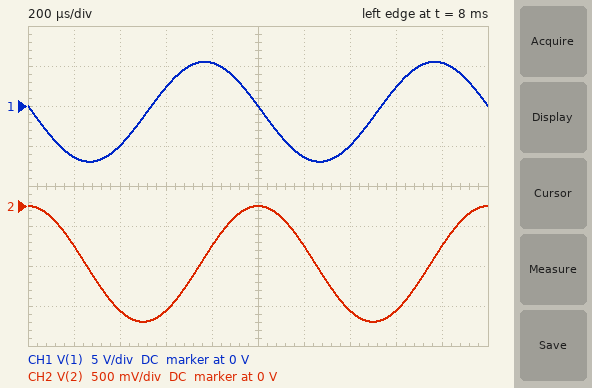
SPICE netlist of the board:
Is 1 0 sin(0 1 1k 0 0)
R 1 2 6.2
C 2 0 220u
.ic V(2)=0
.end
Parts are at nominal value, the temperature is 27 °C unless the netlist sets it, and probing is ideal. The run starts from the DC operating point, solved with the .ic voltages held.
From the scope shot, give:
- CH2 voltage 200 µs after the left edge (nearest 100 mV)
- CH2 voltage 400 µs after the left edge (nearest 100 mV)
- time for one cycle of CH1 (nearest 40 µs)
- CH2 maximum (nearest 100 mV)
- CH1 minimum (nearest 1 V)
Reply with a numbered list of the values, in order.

1. -500 mV
2. -1.3 V
3. 1.00 ms
4. 0 V
5. -7 V
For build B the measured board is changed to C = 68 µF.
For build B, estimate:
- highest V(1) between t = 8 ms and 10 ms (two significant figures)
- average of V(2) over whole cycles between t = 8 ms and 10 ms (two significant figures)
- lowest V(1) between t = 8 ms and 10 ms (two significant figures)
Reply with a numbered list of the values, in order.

1. 4.3 V
2. -2.3 V
3. -9.0 V
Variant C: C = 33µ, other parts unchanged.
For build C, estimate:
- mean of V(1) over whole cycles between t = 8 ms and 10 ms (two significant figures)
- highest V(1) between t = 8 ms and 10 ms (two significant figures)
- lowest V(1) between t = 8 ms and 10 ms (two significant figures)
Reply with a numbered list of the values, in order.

1. -4.8 V
2. 3.0 V
3. -13 V
